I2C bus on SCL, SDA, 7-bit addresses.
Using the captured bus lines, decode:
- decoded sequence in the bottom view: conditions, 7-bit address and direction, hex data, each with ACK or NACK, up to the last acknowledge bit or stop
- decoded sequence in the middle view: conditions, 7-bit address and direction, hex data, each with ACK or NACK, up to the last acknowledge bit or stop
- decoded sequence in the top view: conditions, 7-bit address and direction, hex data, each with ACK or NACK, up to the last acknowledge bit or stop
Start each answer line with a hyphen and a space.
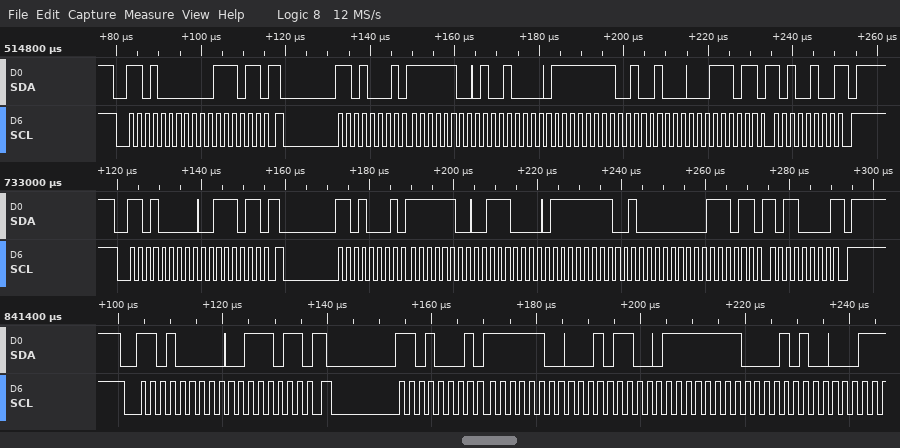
- start, address 68 write ACK, 3B ACK, repeated start, address 68 read ACK, FC ACK, 2C ACK, FF ACK, 14 ACK
- start, address 68 write ACK, 3B ACK, repeated start, address 68 read ACK, FC ACK, 70 ACK, FF ACK, 40 ACK, 3B ACK, B0 NACK, stop
- start, address 68 write ACK, 3B ACK, repeated start, address 68 read ACK, FC ACK, 90 ACK, FF ACK, 48 ACK, 3B ACK, A4 NACK, stop
